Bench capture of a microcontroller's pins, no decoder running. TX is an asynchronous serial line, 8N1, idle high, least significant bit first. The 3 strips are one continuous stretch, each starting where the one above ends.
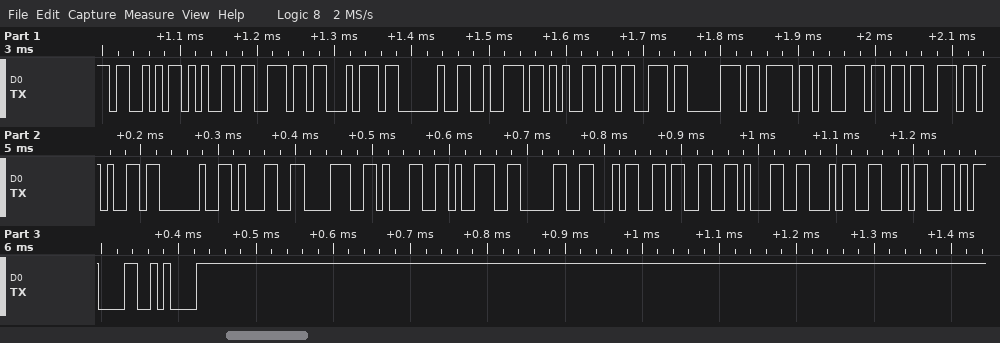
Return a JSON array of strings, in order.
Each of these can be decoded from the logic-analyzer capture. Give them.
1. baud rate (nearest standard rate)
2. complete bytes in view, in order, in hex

["115200 baud", "53 65 6E 74 20 72 65 73 70 6F 6E 73 65 20 31 38 31 39 30 34 33 31 34 34 0D 0A"]
